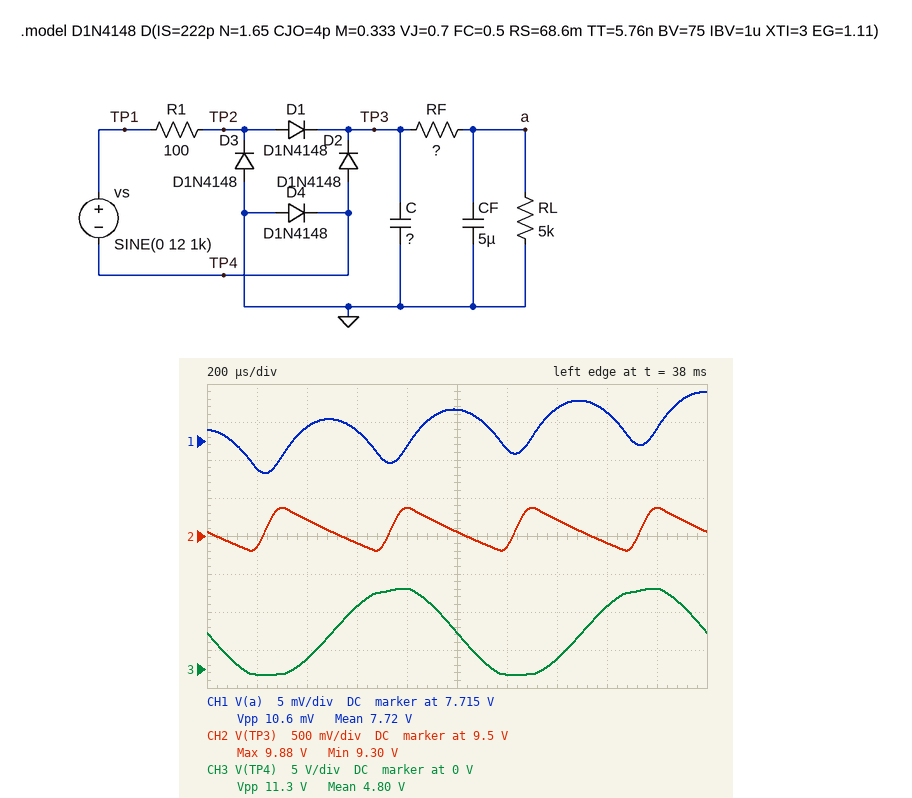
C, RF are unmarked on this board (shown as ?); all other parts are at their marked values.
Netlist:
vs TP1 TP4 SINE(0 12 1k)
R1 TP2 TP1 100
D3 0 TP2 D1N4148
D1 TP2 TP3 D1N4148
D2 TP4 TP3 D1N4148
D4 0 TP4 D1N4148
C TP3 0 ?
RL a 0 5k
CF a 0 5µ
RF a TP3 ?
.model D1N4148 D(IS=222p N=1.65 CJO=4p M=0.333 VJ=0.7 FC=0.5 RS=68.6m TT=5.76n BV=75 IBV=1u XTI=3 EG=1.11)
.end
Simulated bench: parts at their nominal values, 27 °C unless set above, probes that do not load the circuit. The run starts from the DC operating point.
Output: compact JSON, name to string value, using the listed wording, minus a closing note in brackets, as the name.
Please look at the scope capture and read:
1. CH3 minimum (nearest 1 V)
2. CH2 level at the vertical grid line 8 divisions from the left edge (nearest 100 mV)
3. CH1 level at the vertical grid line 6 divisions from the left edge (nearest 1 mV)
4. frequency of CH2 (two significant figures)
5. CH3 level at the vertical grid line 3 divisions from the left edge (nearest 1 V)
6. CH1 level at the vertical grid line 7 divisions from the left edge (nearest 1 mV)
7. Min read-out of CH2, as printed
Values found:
{"CH3 minimum": "-1 V", "CH2 level at the vertical grid line 8 divisions from the left edge": "9.4 V", "CH1 level at the vertical grid line 6 divisions from the left edge": "7.714 V", "frequency of CH2": "2.0 kHz", "CH3 level at the vertical grid line 3 divisions from the left edge": "8 V", "CH1 level at the vertical grid line 7 divisions from the left edge": "7.719 V", "Min read-out of CH2, as printed": "9.30 V"}
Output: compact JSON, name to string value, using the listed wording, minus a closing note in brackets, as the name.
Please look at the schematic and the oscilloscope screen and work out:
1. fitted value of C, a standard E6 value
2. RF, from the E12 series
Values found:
{"fitted value of C, a standard E6 value": "1 µF", "RF, from the E12 series": "1.2 kΩ"}
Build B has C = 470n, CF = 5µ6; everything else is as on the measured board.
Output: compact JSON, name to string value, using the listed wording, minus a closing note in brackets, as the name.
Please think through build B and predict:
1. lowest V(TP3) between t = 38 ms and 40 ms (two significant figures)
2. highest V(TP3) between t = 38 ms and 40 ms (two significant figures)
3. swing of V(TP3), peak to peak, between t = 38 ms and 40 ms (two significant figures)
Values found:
{"lowest V(TP3) between t = 38 ms and 40 ms": "8.9 V", "highest V(TP3) between t = 38 ms and 40 ms": "10 V", "swing of V(TP3), peak to peak, between t = 38 ms and 40 ms": "1.2 V"}
